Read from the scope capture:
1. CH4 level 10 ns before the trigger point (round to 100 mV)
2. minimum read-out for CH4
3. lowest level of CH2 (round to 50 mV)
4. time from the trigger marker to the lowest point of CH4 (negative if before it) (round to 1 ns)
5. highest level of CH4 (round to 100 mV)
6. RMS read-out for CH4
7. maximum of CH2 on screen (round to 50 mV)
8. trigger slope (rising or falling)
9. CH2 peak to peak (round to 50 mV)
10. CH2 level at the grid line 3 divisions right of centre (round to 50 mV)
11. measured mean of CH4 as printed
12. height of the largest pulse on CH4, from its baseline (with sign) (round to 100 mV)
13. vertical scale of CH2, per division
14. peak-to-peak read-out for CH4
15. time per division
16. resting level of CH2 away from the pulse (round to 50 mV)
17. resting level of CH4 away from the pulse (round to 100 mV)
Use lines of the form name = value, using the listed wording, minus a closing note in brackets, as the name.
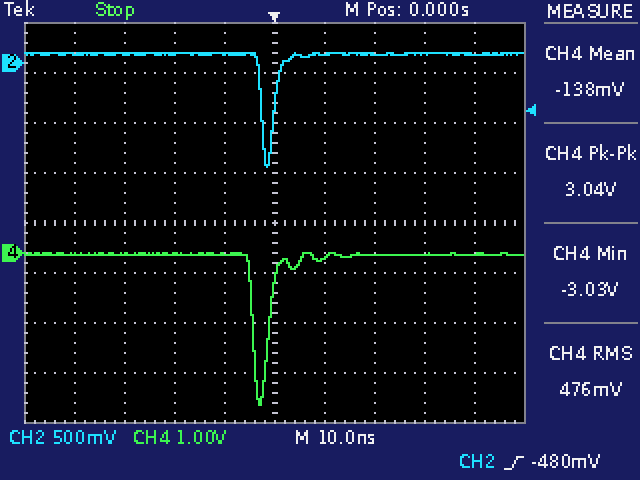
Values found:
CH4 level 10 ns before the trigger point = 0.0 V
minimum read-out for CH4 = -3.03 V
lowest level of CH2 = -1.05 V
time from the trigger marker to the lowest point of CH4 (negative if before it) = -3 ns
highest level of CH4 = 0.0 V
RMS read-out for CH4 = 476 mV
maximum of CH2 on screen = 100 mV
trigger slope = rising
CH2 peak to peak = 1.15 V
CH2 level at the grid line 3 divisions right of centre = 100 mV
measured mean of CH4 as printed = -138 mV
height of the largest pulse on CH4, from its baseline (with sign) = -3.0 V
vertical scale of CH2, per division = 500 mV
peak-to-peak read-out for CH4 = 3.04 V
time per division = 10 ns
resting level of CH2 away from the pulse = 100 mV
resting level of CH4 away from the pulse = 0.0 V
